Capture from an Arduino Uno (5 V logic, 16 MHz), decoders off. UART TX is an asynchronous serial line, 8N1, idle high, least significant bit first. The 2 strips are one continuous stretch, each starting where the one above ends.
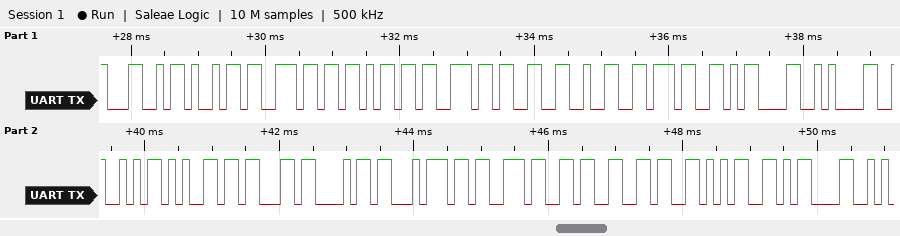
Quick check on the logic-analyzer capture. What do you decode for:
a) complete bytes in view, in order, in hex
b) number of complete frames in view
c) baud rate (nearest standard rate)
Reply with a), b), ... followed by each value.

a) 0x4C 0x69 0x6E 0x6B 0x73 0x33 0x32 0x37 0x0D 0x0A 0x52 0x65 0x63 0x68 0x74 0x73 0x36 0x36 0x35 0x0D
b) 20
c) 9600 baud
